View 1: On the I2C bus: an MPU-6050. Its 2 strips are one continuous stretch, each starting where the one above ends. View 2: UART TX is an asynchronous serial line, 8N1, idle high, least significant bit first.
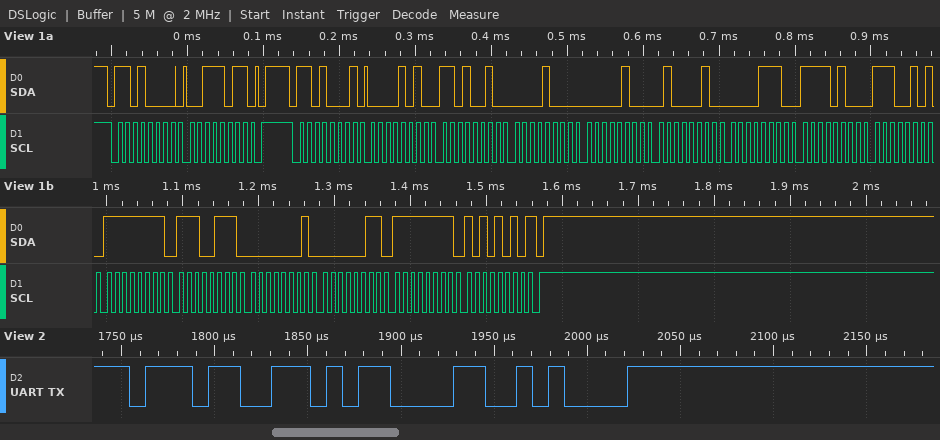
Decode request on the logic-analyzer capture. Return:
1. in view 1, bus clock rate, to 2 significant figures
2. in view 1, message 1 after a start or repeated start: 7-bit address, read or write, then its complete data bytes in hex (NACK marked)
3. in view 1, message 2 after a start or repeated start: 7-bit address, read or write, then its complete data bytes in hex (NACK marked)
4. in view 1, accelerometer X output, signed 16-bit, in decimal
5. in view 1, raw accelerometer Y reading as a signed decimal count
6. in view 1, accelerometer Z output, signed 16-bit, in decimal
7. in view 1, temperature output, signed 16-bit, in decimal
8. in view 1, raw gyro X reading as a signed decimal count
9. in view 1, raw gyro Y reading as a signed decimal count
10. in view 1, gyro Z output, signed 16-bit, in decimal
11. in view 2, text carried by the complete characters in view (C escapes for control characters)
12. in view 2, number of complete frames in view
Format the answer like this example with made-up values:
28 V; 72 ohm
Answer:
100 kHz; 0x68 write: 3B; 0x68 read: 0A D2 08 04 42 0E F4 E5 FF E7 01 03 FF AA NACK; 2770; 2052; 16910; -2843; -25; 259; -86; "7\r\n"; 3
